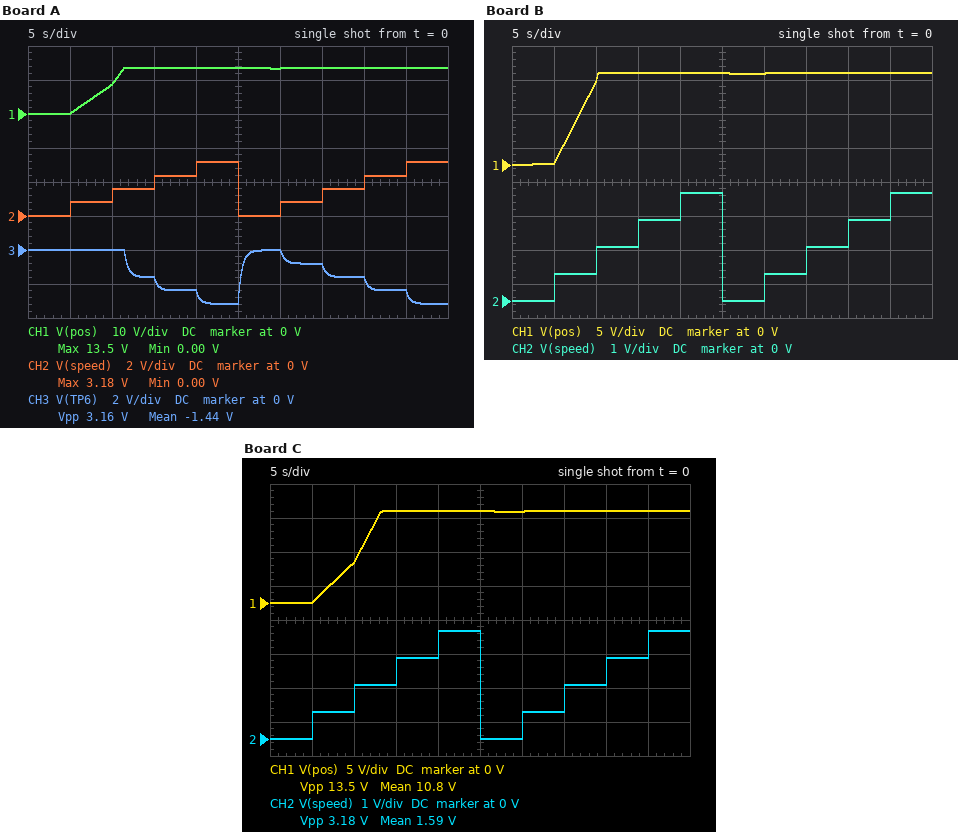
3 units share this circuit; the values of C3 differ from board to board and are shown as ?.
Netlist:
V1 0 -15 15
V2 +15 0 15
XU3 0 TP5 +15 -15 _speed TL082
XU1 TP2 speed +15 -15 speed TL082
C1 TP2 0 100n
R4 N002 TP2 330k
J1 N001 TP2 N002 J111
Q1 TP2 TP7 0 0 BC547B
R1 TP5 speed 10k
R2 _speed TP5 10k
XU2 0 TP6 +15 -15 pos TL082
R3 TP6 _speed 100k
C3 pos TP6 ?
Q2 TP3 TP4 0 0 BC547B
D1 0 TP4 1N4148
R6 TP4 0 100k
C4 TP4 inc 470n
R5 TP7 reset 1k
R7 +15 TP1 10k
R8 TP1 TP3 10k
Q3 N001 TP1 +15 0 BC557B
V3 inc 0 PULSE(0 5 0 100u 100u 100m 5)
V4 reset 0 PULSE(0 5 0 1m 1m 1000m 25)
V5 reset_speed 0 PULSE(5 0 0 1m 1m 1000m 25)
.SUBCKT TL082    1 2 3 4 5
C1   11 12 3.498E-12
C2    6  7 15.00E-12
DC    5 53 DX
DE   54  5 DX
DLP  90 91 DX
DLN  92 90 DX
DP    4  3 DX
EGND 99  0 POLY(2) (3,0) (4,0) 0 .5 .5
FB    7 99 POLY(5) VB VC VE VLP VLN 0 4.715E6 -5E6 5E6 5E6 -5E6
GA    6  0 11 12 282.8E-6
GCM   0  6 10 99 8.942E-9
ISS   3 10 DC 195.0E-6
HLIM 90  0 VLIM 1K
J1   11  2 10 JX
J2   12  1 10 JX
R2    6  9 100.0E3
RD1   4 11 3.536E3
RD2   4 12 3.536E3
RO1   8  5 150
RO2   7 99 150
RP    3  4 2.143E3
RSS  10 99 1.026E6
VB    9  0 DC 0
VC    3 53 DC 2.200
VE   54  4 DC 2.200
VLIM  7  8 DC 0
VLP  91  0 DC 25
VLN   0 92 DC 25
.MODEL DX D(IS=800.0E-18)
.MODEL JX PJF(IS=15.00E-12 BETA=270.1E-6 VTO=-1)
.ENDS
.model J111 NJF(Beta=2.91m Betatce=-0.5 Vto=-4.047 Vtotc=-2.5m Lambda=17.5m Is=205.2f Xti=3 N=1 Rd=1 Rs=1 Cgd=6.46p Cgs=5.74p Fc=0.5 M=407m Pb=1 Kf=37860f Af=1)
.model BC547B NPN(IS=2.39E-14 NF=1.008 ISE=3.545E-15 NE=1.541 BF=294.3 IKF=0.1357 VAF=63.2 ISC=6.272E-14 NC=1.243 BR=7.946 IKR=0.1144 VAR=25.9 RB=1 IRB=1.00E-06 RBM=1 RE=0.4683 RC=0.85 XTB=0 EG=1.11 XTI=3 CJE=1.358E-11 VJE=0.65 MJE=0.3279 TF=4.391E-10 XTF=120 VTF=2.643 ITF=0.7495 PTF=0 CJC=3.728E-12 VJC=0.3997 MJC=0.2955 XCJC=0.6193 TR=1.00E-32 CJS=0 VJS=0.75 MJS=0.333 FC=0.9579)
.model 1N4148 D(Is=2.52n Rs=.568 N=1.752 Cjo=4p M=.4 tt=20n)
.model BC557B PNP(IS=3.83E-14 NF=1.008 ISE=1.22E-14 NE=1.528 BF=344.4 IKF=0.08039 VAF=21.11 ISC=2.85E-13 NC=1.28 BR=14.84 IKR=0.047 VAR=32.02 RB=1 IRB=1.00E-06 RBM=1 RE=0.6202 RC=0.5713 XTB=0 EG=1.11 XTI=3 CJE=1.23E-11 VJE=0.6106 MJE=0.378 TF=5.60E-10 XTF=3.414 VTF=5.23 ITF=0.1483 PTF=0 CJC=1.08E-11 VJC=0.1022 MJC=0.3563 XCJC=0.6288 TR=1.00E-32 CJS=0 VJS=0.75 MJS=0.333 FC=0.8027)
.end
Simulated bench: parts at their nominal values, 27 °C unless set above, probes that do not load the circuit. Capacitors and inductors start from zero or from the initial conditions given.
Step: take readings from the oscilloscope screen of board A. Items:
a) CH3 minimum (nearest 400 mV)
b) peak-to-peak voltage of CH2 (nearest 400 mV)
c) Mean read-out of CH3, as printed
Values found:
-3.2 V
3.2 V
-1.44 V
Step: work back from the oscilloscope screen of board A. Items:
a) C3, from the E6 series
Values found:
4.7 µF
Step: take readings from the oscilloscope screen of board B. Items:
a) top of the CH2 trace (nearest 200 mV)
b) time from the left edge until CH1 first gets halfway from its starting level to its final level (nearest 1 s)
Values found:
3.2 V
8 s
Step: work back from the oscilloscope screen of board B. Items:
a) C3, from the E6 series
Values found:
3.3 µF
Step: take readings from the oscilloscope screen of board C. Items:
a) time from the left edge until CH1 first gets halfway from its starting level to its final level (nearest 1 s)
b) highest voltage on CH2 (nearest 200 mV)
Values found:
10 s
3.2 V
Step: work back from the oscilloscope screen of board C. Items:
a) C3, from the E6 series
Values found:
6.8 µF
